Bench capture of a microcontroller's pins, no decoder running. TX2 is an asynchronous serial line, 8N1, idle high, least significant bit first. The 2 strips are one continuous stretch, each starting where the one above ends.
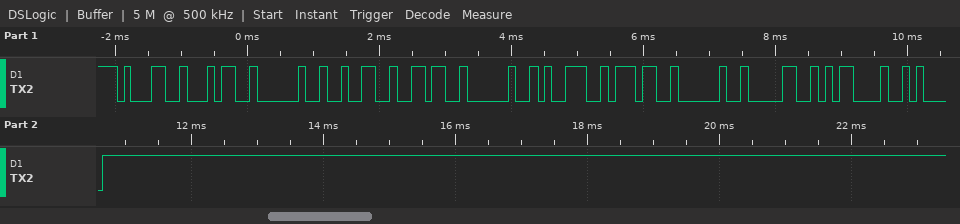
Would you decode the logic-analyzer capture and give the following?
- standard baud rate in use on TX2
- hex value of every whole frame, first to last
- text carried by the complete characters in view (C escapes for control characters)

9600 baud
31 34 20 32 36 20 39 37 20 30 0D 0A
"14 26 97 0\r\n"
